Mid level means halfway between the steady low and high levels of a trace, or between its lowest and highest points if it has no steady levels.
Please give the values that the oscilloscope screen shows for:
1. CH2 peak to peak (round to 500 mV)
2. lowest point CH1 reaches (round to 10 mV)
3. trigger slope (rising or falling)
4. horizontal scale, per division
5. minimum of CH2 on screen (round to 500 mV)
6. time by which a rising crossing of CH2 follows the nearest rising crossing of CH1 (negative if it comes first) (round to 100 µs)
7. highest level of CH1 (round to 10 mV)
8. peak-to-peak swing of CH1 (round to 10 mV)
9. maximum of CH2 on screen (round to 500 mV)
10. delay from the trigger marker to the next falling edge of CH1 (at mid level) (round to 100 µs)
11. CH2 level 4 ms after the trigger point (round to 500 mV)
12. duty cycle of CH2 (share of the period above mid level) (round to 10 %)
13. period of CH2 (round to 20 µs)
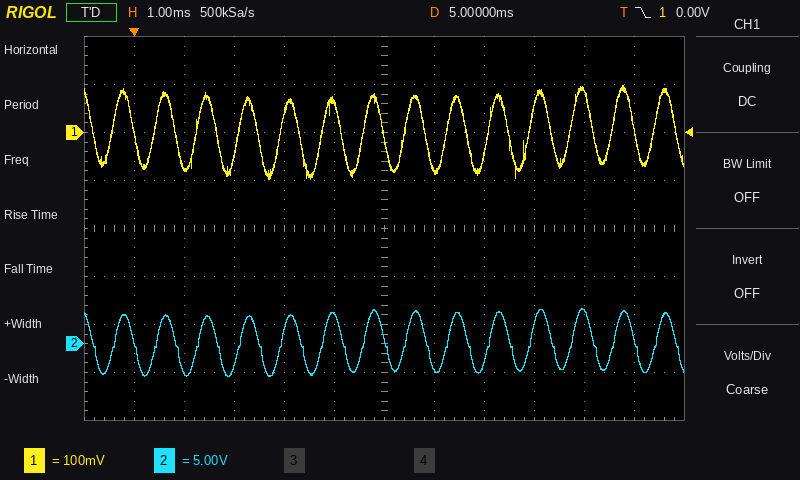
7.0 V
-100 mV
falling
1 ms
-3.5 V
0.0 ms
100 mV
200 mV
3.5 V
800 µs
3.0 V
50 %
840 µs
